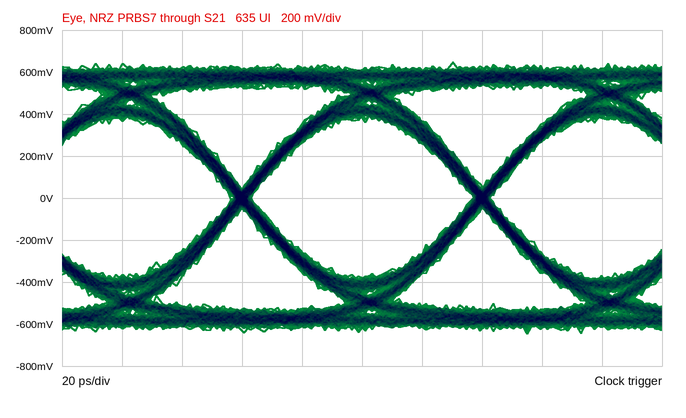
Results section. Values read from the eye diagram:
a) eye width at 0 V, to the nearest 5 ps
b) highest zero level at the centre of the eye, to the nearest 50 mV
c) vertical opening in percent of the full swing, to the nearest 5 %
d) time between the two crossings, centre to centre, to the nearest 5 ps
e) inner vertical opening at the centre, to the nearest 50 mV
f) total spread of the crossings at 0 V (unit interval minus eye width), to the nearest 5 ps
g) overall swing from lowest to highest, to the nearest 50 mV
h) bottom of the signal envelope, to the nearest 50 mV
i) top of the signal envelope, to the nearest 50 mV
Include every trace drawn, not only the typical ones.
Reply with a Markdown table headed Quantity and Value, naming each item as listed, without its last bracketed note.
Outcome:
| Quantity | Value |
|---|---|
| eye width at 0 V, to the nearest 5 ps | 75 ps |
| highest zero level at the centre of the eye, to the nearest 50 mV | -400 mV |
| vertical opening in percent of the full swing, to the nearest 5 % | 60 % |
| time between the two crossings, centre to centre, to the nearest 5 ps | 80 ps |
| inner vertical opening at the centre, to the nearest 50 mV | 750 mV |
| total spread of the crossings at 0 V (unit interval minus eye width), to the nearest 5 ps | 5 ps |
| overall swing from lowest to highest, to the nearest 50 mV | 1.30 V |
| bottom of the signal envelope, to the nearest 50 mV | -650 mV |
| top of the signal envelope, to the nearest 50 mV | 650 mV |
